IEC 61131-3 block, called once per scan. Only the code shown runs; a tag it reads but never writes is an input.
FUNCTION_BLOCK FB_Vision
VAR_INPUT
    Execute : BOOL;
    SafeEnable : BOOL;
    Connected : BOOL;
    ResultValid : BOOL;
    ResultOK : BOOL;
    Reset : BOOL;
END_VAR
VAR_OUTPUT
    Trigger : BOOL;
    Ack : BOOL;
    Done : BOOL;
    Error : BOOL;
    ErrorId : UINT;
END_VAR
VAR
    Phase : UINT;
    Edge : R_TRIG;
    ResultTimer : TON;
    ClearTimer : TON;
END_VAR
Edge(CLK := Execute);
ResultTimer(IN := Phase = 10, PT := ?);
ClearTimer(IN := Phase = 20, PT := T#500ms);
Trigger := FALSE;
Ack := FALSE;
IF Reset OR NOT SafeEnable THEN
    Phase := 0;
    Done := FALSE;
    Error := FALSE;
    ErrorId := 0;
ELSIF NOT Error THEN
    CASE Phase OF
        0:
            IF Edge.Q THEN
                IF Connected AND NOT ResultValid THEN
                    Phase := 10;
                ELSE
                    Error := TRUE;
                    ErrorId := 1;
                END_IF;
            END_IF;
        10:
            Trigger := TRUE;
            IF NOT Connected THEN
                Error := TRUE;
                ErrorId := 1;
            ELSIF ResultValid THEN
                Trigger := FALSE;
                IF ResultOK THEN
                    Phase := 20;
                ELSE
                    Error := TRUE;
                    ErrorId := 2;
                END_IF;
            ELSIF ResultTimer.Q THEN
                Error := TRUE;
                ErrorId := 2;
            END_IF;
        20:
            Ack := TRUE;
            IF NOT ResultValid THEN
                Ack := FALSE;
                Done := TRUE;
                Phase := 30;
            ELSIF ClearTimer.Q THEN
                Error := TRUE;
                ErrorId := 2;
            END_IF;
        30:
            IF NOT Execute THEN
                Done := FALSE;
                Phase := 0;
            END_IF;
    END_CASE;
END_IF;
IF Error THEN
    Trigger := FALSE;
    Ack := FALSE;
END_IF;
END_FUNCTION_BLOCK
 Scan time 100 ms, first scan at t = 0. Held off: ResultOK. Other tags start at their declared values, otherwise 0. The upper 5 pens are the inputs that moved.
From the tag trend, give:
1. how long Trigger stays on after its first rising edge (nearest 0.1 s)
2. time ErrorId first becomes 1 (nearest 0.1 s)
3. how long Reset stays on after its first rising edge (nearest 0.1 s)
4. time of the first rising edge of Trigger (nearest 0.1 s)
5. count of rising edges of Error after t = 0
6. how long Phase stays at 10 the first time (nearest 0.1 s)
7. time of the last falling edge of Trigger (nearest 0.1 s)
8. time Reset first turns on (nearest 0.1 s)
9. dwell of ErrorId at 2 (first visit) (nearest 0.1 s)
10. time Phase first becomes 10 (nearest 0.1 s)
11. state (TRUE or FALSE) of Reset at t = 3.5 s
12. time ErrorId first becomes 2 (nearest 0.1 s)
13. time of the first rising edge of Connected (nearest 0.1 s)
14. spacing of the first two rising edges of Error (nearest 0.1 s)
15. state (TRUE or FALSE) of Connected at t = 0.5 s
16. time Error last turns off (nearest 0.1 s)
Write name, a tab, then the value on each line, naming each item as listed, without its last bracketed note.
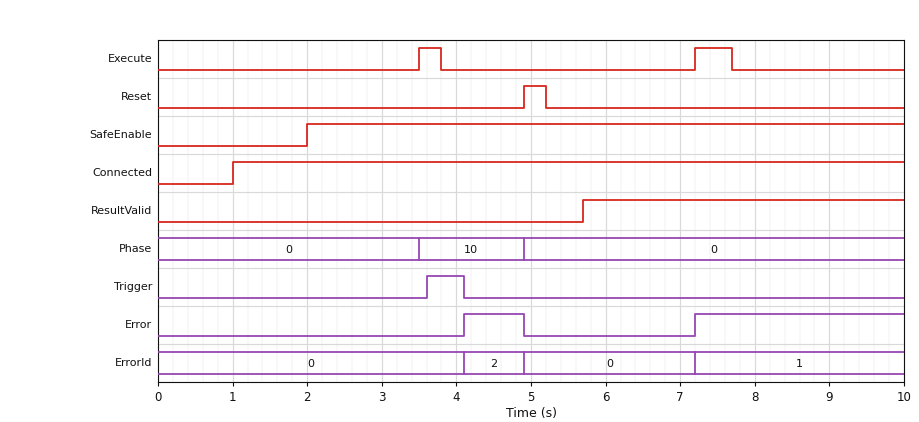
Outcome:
how long Trigger stays on after its first rising edge	0.5 s
time ErrorId first becomes 1	7.2 s
how long Reset stays on after its first rising edge	0.3 s
time of the first rising edge of Trigger	3.6 s
count of rising edges of Error after t = 0	2
how long Phase stays at 10 the first time	1.4 s
time of the last falling edge of Trigger	4.1 s
time Reset first turns on	4.9 s
dwell of ErrorId at 2 (first visit)	0.8 s
time Phase first becomes 10	3.5 s
state (TRUE or FALSE) of Reset at t = 3.5 s	FALSE
time ErrorId first becomes 2	4.1 s
time of the first rising edge of Connected	1.0 s
spacing of the first two rising edges of Error	3.1 s
state (TRUE or FALSE) of Connected at t = 0.5 s	FALSE
time Error last turns off	4.9 s
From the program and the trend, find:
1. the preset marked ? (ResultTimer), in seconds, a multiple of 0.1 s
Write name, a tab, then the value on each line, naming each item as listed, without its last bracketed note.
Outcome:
the preset marked ? (ResultTimer), in seconds, a multiple of 0.1 s	0.5 s
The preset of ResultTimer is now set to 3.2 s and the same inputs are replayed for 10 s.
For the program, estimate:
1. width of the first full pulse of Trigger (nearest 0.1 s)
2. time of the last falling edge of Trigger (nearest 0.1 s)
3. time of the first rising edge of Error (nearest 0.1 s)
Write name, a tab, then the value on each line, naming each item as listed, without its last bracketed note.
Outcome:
width of the first full pulse of Trigger	1.3 s
time of the last falling edge of Trigger	4.9 s
time of the first rising edge of Error	7.2 s
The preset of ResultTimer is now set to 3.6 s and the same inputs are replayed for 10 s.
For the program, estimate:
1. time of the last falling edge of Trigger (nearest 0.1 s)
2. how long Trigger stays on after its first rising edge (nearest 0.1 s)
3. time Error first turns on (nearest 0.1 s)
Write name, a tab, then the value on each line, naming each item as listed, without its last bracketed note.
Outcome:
time of the last falling edge of Trigger	4.9 s
how long Trigger stays on after its first rising edge	1.3 s
time Error first turns on	7.2 s
